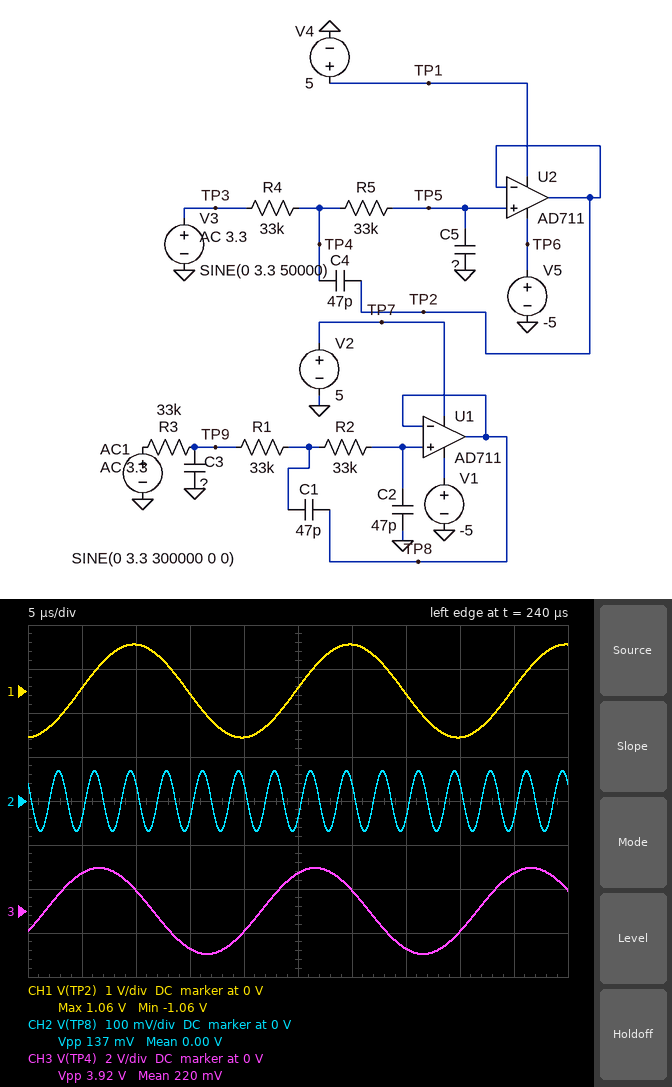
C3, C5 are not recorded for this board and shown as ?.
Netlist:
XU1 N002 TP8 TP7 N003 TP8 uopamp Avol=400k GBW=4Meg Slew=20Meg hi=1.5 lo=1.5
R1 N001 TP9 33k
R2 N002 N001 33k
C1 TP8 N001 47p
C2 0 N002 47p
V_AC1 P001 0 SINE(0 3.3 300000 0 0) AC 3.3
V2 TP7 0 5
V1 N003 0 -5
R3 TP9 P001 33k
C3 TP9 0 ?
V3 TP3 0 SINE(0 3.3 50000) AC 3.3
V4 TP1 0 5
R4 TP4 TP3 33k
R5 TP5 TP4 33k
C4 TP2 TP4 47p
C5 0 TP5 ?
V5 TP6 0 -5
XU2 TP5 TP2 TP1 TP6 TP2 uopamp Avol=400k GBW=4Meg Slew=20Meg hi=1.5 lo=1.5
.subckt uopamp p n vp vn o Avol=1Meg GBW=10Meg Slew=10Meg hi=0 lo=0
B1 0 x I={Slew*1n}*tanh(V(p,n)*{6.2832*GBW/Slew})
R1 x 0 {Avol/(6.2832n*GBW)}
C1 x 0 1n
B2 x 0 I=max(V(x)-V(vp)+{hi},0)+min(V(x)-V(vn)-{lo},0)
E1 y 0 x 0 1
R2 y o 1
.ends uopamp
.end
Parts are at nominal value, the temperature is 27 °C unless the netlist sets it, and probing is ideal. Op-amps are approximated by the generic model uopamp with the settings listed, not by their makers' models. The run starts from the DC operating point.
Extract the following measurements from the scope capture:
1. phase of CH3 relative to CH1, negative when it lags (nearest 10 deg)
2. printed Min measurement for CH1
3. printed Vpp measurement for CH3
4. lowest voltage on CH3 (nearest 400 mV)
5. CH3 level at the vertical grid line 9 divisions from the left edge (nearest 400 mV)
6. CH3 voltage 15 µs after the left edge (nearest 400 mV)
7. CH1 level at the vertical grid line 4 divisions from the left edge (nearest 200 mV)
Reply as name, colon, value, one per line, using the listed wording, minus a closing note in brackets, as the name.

phase of CH3 relative to CH1, negative when it lags: 60 deg
printed Min measurement for CH1: -1.06 V
printed Vpp measurement for CH3: 3.92 V
lowest voltage on CH3: -2.0 V
CH3 level at the vertical grid line 9 divisions from the left edge: 1.6 V
CH3 voltage 15 µs after the left edge: -1.6 V
CH1 level at the vertical grid line 4 divisions from the left edge: -1.0 V
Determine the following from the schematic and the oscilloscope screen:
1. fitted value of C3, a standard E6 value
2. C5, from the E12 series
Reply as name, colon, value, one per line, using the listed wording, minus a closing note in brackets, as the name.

fitted value of C3, a standard E6 value: 68 pF
C5, from the E12 series: 150 pF
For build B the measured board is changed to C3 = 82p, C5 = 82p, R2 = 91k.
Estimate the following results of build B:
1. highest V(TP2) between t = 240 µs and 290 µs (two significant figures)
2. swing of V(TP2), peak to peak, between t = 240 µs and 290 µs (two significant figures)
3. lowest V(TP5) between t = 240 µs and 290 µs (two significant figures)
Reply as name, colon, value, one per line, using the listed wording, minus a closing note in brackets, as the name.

highest V(TP2) between t = 240 µs and 290 µs: 1.8 V
swing of V(TP2), peak to peak, between t = 240 µs and 290 µs: 3.7 V
lowest V(TP5) between t = 240 µs and 290 µs: -1.8 V
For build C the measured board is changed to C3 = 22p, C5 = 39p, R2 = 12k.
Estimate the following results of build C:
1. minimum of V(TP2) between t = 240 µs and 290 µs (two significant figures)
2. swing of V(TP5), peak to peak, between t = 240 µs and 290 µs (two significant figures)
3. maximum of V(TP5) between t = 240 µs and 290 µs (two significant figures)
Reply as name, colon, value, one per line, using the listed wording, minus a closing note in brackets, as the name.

minimum of V(TP2) between t = 240 µs and 290 µs: -2.9 V
swing of V(TP5), peak to peak, between t = 240 µs and 290 µs: 5.8 V
maximum of V(TP5) between t = 240 µs and 290 µs: 2.9 V
